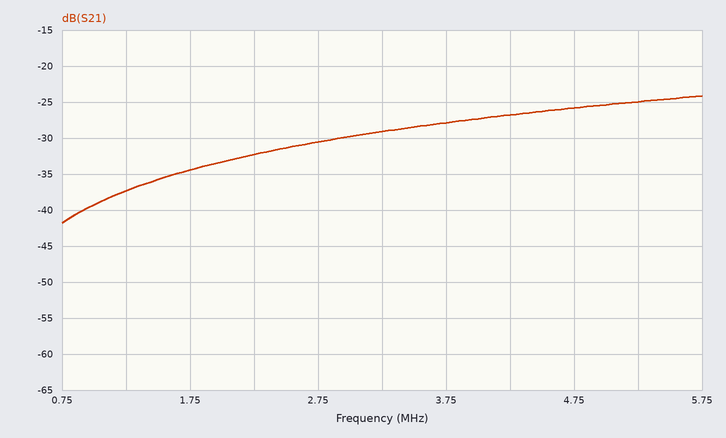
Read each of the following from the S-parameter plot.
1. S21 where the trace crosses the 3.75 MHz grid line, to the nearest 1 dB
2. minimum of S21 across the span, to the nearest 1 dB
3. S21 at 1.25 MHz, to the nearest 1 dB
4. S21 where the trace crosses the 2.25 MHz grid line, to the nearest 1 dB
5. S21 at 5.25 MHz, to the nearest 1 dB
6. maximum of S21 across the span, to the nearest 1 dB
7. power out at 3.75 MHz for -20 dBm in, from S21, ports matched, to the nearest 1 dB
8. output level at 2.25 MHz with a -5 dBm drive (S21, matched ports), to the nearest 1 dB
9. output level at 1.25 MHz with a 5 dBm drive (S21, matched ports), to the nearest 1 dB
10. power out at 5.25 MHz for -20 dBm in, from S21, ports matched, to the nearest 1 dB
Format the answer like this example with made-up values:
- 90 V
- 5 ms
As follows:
- -28 dB
- -42 dB
- -37 dB
- -32 dB
- -25 dB
- -24 dB
- -48 dBm
- -37 dBm
- -32 dBm
- -45 dBm
